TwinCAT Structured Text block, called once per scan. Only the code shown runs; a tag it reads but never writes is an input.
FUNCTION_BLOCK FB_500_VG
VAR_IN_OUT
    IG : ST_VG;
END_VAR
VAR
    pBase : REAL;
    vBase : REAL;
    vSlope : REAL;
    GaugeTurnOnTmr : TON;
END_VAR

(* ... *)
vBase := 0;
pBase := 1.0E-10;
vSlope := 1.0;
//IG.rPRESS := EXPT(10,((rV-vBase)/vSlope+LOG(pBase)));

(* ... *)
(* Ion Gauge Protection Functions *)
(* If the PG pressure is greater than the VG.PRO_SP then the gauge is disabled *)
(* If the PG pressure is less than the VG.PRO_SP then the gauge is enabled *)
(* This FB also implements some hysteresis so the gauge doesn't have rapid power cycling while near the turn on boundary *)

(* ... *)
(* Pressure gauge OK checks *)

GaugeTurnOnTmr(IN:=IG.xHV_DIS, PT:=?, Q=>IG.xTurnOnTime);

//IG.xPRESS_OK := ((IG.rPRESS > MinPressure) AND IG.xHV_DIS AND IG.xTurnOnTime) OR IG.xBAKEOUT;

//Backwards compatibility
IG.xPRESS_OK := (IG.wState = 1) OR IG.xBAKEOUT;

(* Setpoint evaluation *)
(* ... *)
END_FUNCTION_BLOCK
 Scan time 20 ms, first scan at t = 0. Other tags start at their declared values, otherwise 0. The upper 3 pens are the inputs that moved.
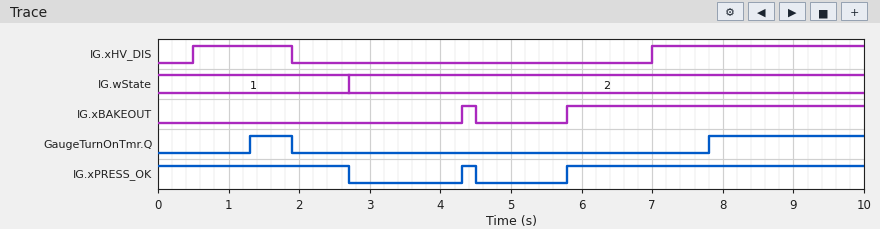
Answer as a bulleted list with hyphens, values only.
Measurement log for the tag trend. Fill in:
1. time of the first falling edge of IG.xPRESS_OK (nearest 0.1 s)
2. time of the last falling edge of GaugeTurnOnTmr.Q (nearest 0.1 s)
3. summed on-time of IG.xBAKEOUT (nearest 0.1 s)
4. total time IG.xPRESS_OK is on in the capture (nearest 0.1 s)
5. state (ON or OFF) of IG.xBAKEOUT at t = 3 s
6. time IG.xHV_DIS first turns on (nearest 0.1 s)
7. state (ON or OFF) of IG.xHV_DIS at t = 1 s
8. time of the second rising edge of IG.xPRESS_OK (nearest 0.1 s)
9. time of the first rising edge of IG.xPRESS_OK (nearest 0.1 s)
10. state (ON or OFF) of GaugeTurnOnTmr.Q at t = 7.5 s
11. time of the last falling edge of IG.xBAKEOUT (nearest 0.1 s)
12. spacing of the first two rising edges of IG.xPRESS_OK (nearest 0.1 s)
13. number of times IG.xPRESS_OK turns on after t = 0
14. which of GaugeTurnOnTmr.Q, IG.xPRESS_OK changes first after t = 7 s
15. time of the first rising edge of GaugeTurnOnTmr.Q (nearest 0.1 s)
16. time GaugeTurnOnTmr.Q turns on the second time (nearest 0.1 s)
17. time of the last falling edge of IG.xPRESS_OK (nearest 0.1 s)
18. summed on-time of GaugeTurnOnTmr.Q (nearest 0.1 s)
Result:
- 2.7 s
- 1.9 s
- 4.4 s
- 7.1 s
- OFF
- 0.5 s
- ON
- 5.8 s
- 4.3 s
- OFF
- 4.5 s
- 1.5 s
- 2
- GaugeTurnOnTmr.Q
- 1.3 s
- 7.8 s
- 4.5 s
- 2.8 s
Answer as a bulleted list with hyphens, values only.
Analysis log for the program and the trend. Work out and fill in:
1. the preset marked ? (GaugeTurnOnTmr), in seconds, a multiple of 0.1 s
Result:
- 0.8 s
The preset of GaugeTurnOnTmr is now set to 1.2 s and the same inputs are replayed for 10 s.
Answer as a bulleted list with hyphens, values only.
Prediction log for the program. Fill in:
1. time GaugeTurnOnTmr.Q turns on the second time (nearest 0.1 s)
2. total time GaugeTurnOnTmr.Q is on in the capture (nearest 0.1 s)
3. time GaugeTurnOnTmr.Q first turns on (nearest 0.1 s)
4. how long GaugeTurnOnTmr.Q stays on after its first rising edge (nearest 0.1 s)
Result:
- 8.2 s
- 2.0 s
- 1.7 s
- 0.2 s
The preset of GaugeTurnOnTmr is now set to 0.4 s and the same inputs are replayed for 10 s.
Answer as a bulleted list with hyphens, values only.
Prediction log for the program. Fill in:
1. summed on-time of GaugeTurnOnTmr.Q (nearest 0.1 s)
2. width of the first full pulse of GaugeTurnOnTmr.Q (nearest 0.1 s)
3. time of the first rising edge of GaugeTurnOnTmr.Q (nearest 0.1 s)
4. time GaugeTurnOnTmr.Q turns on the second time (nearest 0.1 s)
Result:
- 3.6 s
- 1.0 s
- 0.9 s
- 7.4 s
